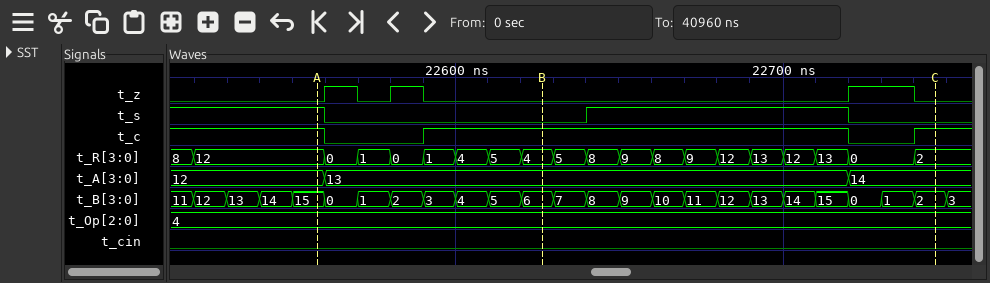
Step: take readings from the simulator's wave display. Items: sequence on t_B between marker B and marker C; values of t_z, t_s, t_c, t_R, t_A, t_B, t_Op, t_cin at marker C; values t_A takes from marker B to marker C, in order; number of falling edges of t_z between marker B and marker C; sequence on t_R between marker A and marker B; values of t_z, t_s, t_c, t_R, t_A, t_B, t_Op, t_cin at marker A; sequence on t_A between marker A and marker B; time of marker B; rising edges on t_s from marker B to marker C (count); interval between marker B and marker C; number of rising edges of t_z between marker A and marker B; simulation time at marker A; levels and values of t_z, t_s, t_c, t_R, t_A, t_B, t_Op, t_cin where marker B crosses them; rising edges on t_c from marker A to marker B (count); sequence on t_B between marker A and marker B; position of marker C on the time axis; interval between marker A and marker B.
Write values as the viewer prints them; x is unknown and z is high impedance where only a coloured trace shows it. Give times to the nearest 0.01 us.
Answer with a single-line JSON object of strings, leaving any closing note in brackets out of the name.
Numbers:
{"sequence on t_B between marker B and marker C": "6, 7, 8, 9, 10, 11, 12, 13, 14, 15, 0, 1, 2", "values of t_z, t_s, t_c, t_R, t_A, t_B, t_Op, t_cin at marker C": "t_z=0, t_s=0, t_c=1, t_R=2, t_A=14, t_B=2, t_Op=4, t_cin=0", "values t_A takes from marker B to marker C, in order": "13, 14", "number of falling edges of t_z between marker B and marker C": "1", "sequence on t_R between marker A and marker B": "12, 0, 1, 0, 1, 4, 5, 4", "values of t_z, t_s, t_c, t_R, t_A, t_B, t_Op, t_cin at marker A": "t_z=0, t_s=1, t_c=1, t_R=12, t_A=12, t_B=15, t_Op=4, t_cin=0", "sequence on t_A between marker A and marker B": "12, 13", "time of marker B": "22.63 us", "rising edges on t_s from marker B to marker C": "1", "interval between marker B and marker C": "0.12 us", "number of rising edges of t_z between marker A and marker B": "2", "simulation time at marker A": "22.56 us", "levels and values of t_z, t_s, t_c, t_R, t_A, t_B, t_Op, t_cin where marker B crosses them": "t_z=0, t_s=0, t_c=1, t_R=4, t_A=13, t_B=6, t_Op=4, t_cin=0", "rising edges on t_c from marker A to marker B": "1", "sequence on t_B between marker A and marker B": "15, 0, 1, 2, 3, 4, 5, 6", "position of marker C on the time axis": "22.75 us", "interval between marker A and marker B": "0.07 us"}
